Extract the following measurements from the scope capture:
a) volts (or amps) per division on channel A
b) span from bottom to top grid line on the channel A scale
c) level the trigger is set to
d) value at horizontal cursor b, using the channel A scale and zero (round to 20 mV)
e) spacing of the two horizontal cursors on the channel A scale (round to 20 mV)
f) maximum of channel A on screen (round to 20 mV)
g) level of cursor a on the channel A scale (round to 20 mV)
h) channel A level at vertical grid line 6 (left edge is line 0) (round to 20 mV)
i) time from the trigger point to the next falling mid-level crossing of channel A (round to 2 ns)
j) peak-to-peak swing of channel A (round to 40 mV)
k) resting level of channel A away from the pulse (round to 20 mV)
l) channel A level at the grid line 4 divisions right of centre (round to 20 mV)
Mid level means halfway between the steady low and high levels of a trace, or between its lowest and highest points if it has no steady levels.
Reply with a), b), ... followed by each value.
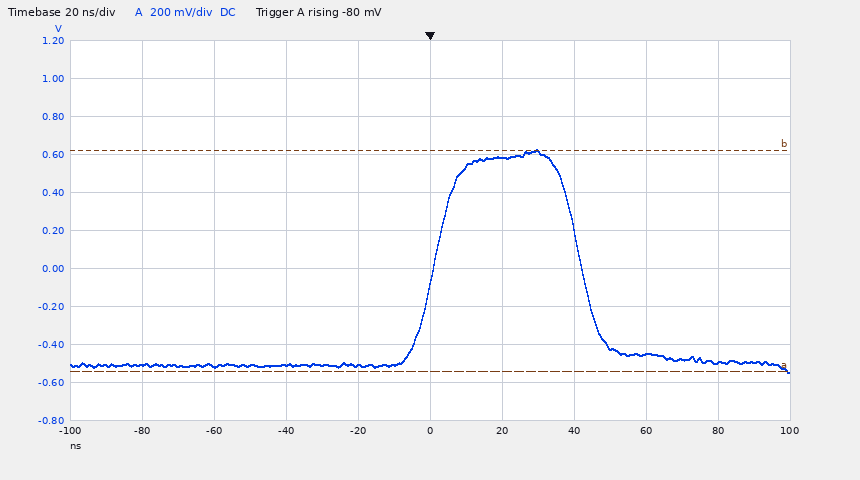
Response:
a) 200 mV
b) 2 V
c) -80 mV
d) 620 mV
e) 1.16 V
f) 620 mV
g) -540 mV
h) 580 mV
i) 42 ns
j) 1.16 V
k) -500 mV
l) -500 mV
